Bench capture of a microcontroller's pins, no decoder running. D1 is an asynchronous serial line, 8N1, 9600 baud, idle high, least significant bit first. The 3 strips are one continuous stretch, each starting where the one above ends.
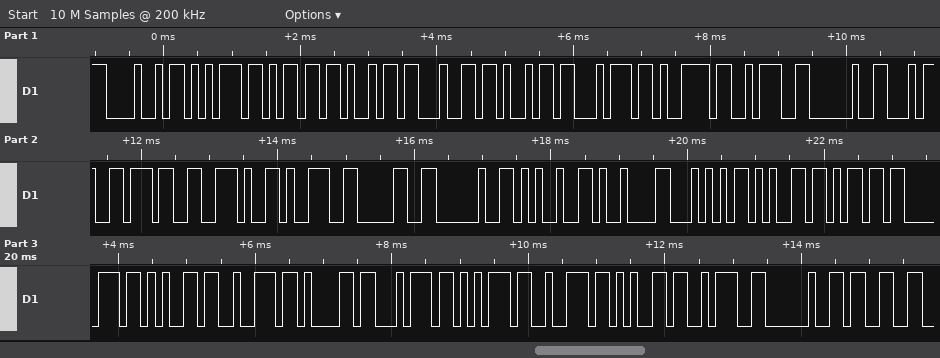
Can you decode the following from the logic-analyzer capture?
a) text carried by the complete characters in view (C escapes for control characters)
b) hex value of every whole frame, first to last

"Humidity: 47.90 %\tTemperature: 3"
48 75 6D 69 64 69 74 79 3A 20 34 37 2E 39 30 20 25 09 54 65 6D 70 65 72 61 74 75 72 65 3A 20 33
